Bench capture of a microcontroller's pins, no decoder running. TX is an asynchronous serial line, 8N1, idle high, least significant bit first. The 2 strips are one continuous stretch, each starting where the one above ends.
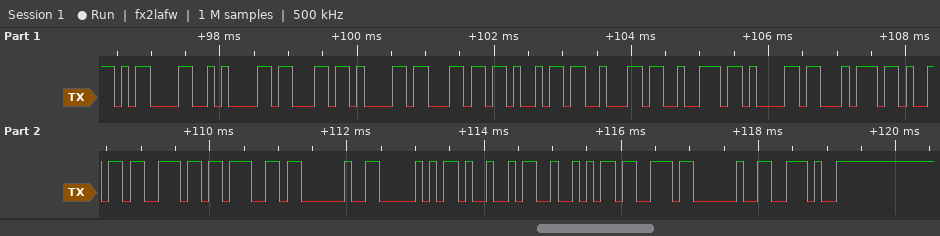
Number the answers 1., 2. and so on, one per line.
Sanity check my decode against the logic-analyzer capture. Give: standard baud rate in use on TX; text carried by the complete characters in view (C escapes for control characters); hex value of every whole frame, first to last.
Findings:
1. 9600 baud
2. "\r\ncalibrating PIRs ."
3. 0D 0A 63 61 6C 69 62 72 61 74 69 6E 67 20 50 49 52 73 20 2E
